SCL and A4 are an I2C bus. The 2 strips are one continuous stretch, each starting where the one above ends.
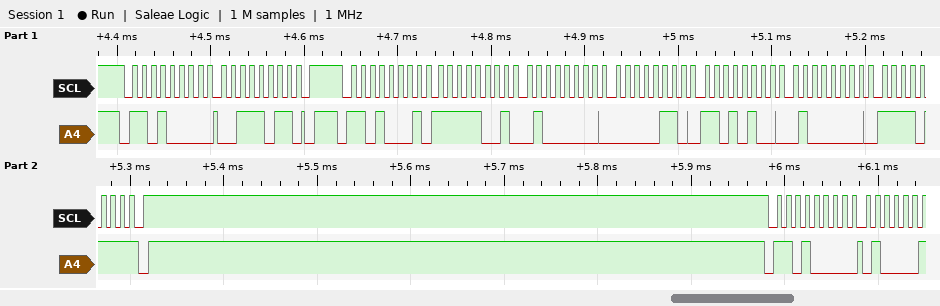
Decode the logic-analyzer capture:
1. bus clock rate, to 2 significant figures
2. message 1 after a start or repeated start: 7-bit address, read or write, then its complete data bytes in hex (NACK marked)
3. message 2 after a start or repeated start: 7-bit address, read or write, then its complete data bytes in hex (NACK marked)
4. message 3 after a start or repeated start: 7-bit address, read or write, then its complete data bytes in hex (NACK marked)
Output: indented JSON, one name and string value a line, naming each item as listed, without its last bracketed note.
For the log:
{
  "bus clock rate, to 2 significant figures": "100 kHz",
  "message 1 after a start or repeated start: 7-bit address, read or write, then its complete data bytes in hex": "0x68 write: 3B",
  "message 2 after a start or repeated start: 7-bit address, read or write, then its complete data bytes in hex": "0x68 read: F9 40 06 D4 40 F7 NACK",
  "message 3 after a start or repeated start: 7-bit address, read or write, then its complete data bytes in hex": "0x68 write"
}
